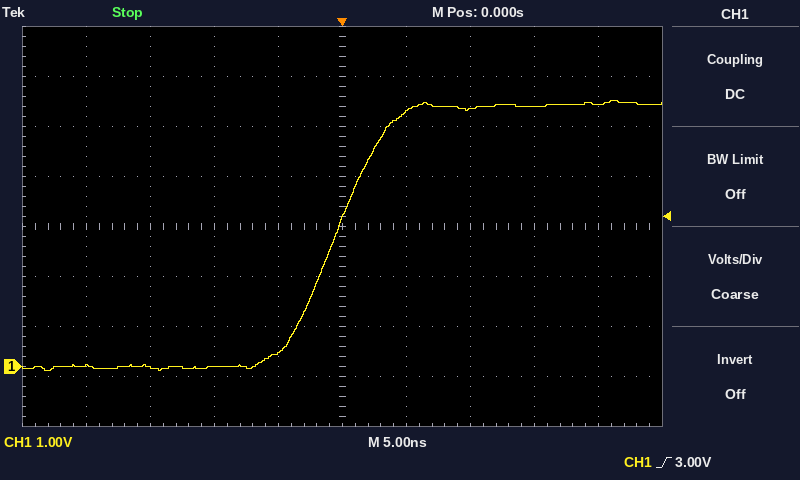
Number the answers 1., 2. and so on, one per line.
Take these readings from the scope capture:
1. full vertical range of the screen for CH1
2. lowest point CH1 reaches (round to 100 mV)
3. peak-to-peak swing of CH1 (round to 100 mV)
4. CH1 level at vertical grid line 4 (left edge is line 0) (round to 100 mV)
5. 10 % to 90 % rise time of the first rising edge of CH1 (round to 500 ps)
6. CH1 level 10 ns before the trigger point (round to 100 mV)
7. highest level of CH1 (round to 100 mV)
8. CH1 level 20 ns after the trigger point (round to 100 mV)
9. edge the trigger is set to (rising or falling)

1. 8 V
2. -100 mV
3. 5.4 V
4. 300 mV
5. 7.5 ns
6. 0.0 V
7. 5.3 V
8. 5.2 V
9. rising
